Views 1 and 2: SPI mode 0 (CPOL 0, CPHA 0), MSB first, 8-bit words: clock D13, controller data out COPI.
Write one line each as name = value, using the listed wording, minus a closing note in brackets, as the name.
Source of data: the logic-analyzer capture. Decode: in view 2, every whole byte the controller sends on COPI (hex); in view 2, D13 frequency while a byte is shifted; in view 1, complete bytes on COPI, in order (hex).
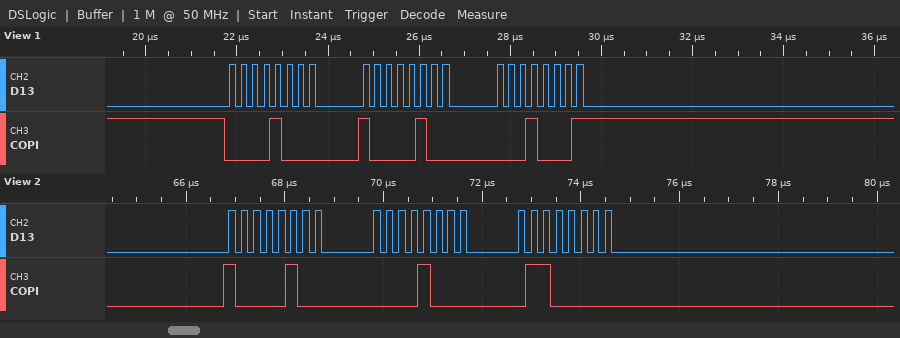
in view 2, every whole byte the controller sends on COPI = 84 08 60
in view 2, D13 frequency while a byte is shifted = 4 MHz
in view 1, complete bytes on COPI, in order = 08 84 11
